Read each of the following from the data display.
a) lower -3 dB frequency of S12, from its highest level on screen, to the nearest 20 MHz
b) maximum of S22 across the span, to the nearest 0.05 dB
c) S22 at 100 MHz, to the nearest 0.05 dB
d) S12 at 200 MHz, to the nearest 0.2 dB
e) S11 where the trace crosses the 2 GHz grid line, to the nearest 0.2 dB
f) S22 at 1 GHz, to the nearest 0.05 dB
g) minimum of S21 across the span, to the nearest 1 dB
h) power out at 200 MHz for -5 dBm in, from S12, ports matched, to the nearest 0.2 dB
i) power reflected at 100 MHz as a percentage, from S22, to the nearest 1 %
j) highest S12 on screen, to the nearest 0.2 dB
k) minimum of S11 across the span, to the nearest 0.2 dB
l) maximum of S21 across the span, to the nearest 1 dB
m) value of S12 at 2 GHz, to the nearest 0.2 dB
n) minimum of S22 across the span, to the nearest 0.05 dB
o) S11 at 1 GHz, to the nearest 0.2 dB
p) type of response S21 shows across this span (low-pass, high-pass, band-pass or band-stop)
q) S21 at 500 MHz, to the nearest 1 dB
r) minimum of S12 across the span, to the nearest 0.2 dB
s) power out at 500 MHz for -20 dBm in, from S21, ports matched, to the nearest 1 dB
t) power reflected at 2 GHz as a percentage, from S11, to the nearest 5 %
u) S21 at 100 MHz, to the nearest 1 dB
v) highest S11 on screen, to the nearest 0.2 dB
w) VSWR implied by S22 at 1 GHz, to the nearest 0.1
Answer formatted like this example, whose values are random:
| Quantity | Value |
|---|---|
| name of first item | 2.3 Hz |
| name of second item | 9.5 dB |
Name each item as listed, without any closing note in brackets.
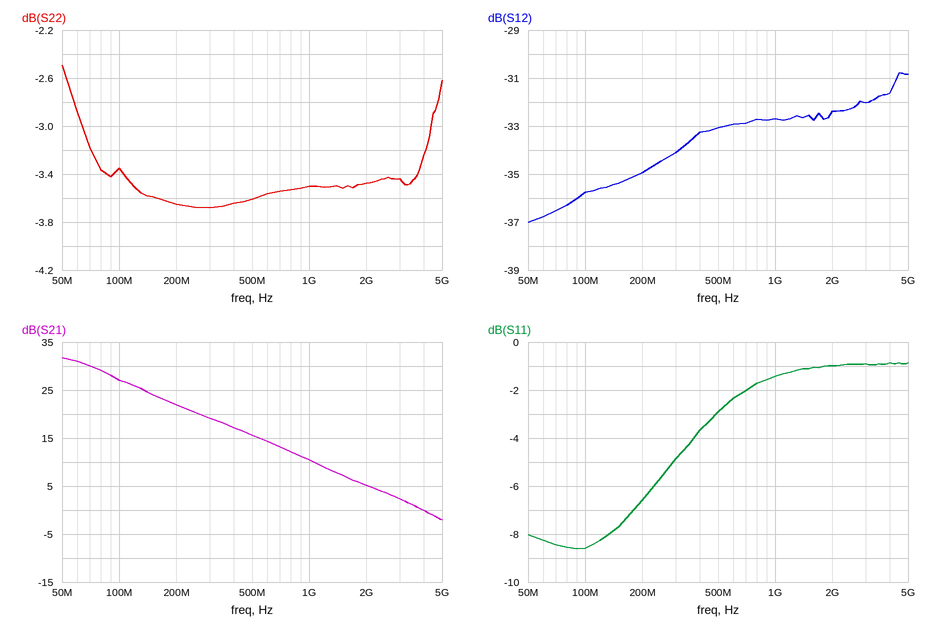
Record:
| Quantity | Value |
|---|---|
| lower -3 dB frequency of S12, from its highest level on screen, to the nearest 20 MHz | 340 MHz |
| maximum of S22 across the span, to the nearest 0.05 dB | -2.50 dB |
| S22 at 100 MHz, to the nearest 0.05 dB | -3.35 dB |
| S12 at 200 MHz, to the nearest 0.2 dB | -35.0 dB |
| S11 where the trace crosses the 2 GHz grid line, to the nearest 0.2 dB | -1.0 dB |
| S22 at 1 GHz, to the nearest 0.05 dB | -3.50 dB |
| minimum of S21 across the span, to the nearest 1 dB | -2 dB |
| power out at 200 MHz for -5 dBm in, from S12, ports matched, to the nearest 0.2 dB | -40.0 dBm |
| power reflected at 100 MHz as a percentage, from S22, to the nearest 1 % | 46 % |
| highest S12 on screen, to the nearest 0.2 dB | -30.8 dB |
| minimum of S11 across the span, to the nearest 0.2 dB | -8.6 dB |
| maximum of S21 across the span, to the nearest 1 dB | 32 dB |
| value of S12 at 2 GHz, to the nearest 0.2 dB | -32.4 dB |
| minimum of S22 across the span, to the nearest 0.05 dB | -3.70 dB |
| S11 at 1 GHz, to the nearest 0.2 dB | -1.4 dB |
| type of response S21 shows across this span | low-pass |
| S21 at 500 MHz, to the nearest 1 dB | 16 dB |
| minimum of S12 across the span, to the nearest 0.2 dB | -37.0 dB |
| power out at 500 MHz for -20 dBm in, from S21, ports matched, to the nearest 1 dB | -4 dBm |
| power reflected at 2 GHz as a percentage, from S11, to the nearest 5 % | 80 % |
| S21 at 100 MHz, to the nearest 1 dB | 27 dB |
| highest S11 on screen, to the nearest 0.2 dB | -0.8 dB |
| VSWR implied by S22 at 1 GHz, to the nearest 0.1 | 5.0 |
